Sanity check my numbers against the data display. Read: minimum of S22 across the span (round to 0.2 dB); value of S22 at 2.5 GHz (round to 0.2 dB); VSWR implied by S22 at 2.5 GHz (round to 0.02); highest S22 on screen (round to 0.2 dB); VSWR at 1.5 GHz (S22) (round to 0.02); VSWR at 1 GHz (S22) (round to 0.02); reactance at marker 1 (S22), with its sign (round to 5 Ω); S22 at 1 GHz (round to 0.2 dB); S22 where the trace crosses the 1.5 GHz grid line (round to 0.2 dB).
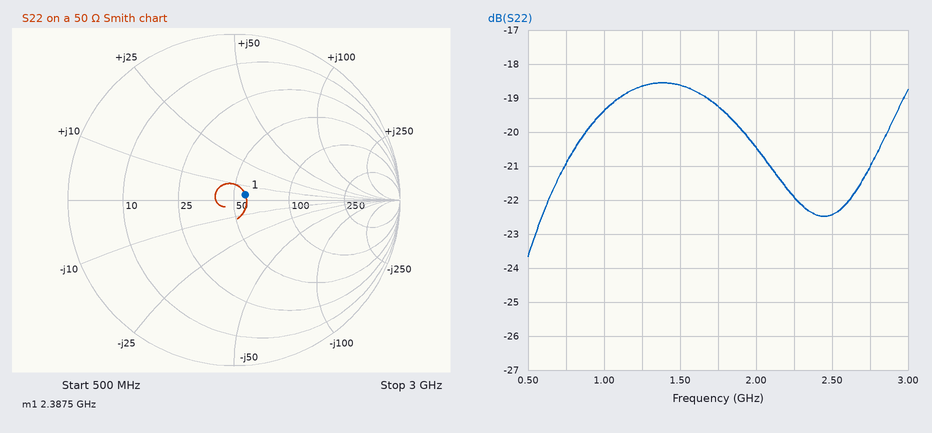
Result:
-23.6 dB
-22.4 dB
1.16
-18.6 dB
1.26
1.24
+5 Ω
-19.4 dB
-18.6 dB
